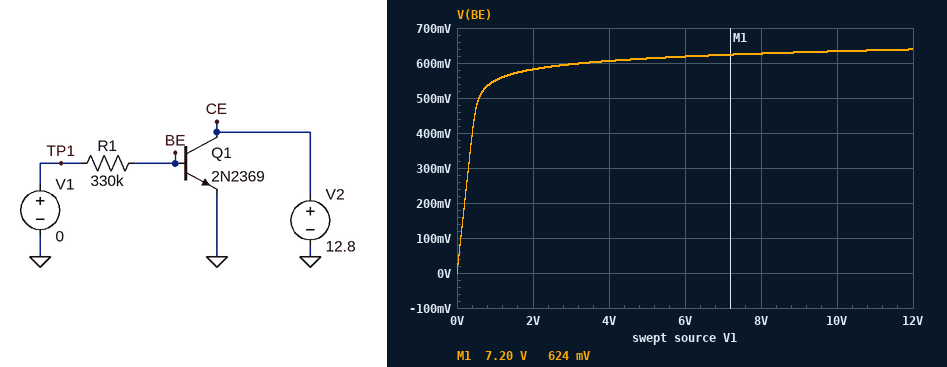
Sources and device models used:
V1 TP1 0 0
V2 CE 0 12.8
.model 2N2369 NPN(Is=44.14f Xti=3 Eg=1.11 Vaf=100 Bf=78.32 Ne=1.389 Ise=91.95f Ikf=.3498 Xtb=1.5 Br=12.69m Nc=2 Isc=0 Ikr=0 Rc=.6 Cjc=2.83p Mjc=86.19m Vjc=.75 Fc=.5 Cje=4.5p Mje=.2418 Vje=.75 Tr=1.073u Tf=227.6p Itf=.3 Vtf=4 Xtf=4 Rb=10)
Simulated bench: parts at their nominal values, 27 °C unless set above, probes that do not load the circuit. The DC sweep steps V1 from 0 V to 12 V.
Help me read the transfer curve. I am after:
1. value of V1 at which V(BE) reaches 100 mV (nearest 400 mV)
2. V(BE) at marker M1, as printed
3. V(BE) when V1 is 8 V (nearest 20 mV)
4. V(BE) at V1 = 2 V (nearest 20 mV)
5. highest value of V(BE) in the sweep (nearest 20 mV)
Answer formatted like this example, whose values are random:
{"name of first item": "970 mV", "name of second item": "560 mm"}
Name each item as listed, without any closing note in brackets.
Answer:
{"value of V1 at which V(BE) reaches 100 mV": "0 V", "V(BE) at marker M1, as printed": "624 mV", "V(BE) when V1 is 8 V": "620 mV", "V(BE) at V1 = 2 V": "580 mV", "highest value of V(BE) in the sweep": "640 mV"}
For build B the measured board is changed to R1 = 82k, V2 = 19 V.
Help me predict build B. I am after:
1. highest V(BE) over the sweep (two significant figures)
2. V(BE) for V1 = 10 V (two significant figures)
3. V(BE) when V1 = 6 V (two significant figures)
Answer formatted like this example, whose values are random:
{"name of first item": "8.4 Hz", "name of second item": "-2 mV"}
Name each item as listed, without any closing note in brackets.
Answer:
{"highest V(BE) over the sweep": "680 mV", "V(BE) for V1 = 10 V": "670 mV", "V(BE) when V1 = 6 V": "660 mV"}
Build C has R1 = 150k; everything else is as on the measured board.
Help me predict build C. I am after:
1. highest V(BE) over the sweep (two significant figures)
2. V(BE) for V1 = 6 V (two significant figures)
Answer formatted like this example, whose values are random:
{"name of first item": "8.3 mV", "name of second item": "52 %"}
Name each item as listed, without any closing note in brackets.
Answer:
{"highest V(BE) over the sweep": "660 mV", "V(BE) for V1 = 6 V": "640 mV"}
